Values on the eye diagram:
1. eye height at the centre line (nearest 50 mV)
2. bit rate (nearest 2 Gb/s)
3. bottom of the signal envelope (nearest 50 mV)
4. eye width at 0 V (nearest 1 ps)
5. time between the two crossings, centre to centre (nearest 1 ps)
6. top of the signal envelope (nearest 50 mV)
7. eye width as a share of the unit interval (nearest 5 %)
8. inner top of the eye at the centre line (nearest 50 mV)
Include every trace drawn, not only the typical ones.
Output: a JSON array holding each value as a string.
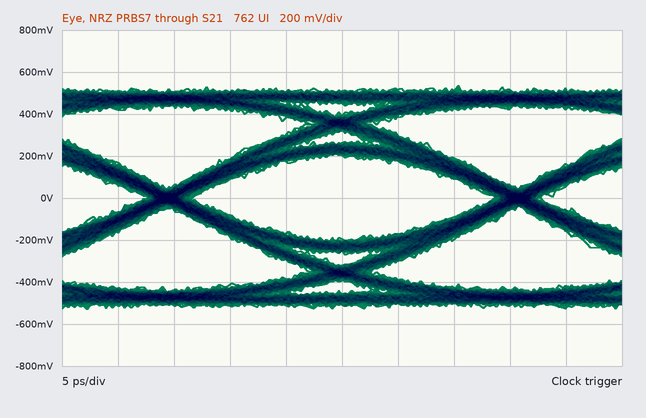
["400 mV", "32 Gb/s", "-550 mV", "27 ps", "31 ps", "550 mV", "85 %", "200 mV"]
